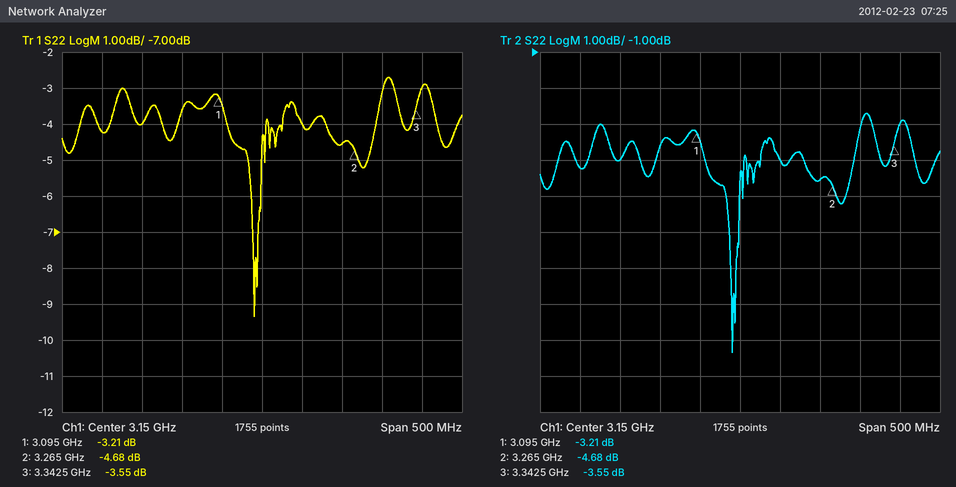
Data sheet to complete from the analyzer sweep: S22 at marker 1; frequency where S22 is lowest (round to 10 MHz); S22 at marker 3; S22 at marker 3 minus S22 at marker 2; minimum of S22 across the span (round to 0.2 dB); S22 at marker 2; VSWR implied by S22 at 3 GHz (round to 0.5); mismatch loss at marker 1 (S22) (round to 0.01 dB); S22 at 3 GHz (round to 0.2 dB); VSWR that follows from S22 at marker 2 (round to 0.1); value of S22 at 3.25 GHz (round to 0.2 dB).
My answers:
-3.21 dB
3.14 GHz
-3.55 dB
1.13 dB
-9.4 dB
-4.68 dB
4.5
2.82 dB
-4.0 dB
3.8
-4.6 dB
